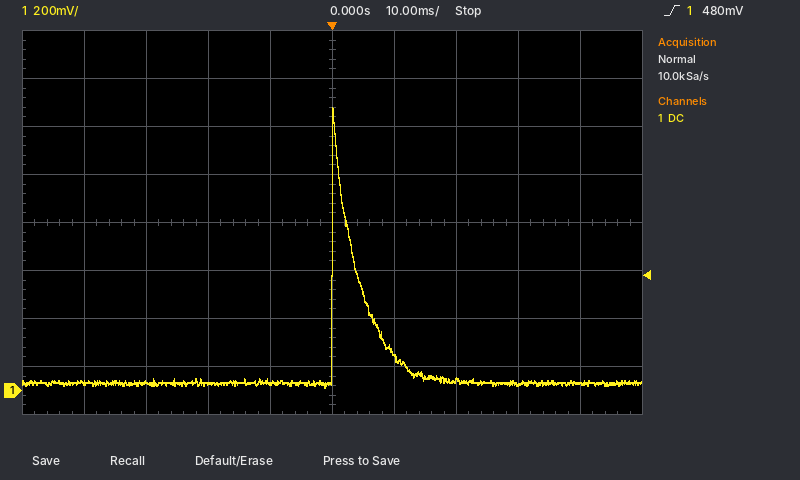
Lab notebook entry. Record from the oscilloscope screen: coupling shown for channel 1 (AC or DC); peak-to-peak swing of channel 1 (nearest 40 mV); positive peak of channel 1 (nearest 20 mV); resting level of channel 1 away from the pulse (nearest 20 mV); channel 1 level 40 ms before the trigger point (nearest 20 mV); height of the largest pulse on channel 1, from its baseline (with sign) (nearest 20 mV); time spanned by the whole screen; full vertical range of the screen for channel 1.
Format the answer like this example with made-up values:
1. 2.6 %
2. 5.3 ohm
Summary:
1. DC
2. 1.16 V
3. 1.18 V
4. 40 mV
5. 40 mV
6. +1.14 V
7. 100 ms
8. 1.6 V
